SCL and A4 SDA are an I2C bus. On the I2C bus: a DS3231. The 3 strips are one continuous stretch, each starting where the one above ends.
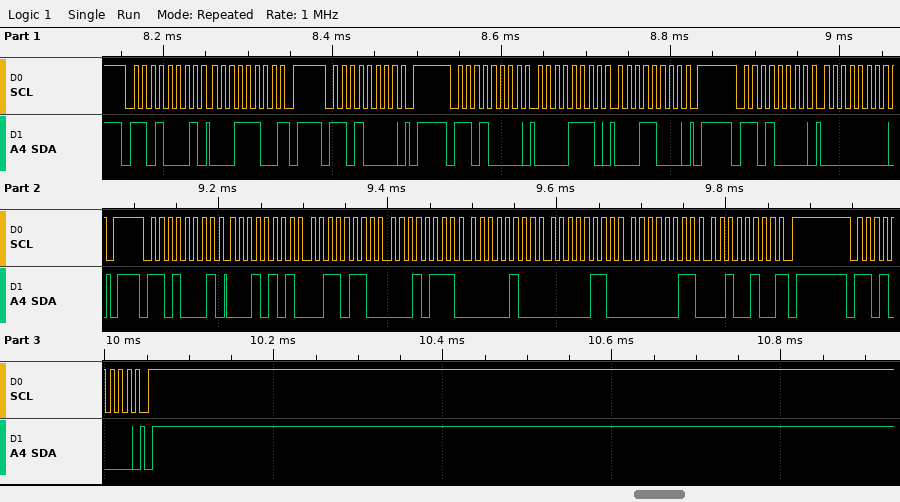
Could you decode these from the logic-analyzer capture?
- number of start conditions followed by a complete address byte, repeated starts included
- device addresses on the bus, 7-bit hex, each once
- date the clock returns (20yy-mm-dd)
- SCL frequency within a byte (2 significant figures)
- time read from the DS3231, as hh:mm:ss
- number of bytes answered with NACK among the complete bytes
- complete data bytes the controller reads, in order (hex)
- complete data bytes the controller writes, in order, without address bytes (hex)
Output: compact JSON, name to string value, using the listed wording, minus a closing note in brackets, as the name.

{"number of start conditions followed by a complete address byte, repeated starts included": "6", "device addresses on the bus, 7-bit hex, each once": "0x68", "date the clock returns": "2024-03-06", "SCL frequency within a byte": "100 kHz", "time read from the DS3231, as hh:mm:ss": "17:36:15", "number of bytes answered with NACK among the complete bytes": "2", "complete data bytes the controller reads, in order": "1C 15 36 17 04 06 03 24", "complete data bytes the controller writes, in order, without address bytes": "0E 18 00"}
